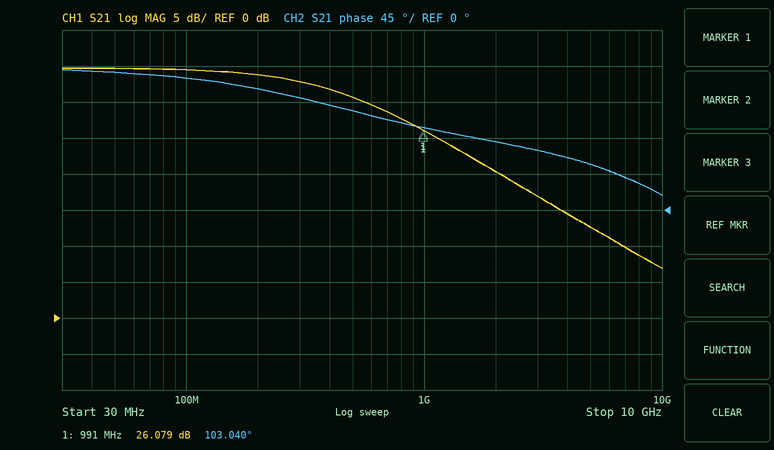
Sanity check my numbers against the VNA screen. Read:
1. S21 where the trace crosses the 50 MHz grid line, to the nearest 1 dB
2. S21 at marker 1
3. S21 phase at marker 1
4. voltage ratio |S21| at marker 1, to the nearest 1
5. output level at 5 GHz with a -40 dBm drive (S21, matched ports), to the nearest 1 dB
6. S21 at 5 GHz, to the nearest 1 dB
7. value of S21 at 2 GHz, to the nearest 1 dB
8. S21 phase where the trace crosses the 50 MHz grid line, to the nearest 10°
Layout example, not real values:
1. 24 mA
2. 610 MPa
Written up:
1. 35 dB
2. 26.079 dB
3. 103.040°
4. 20
5. -27 dBm
6. 13 dB
7. 20 dB
8. 170°
